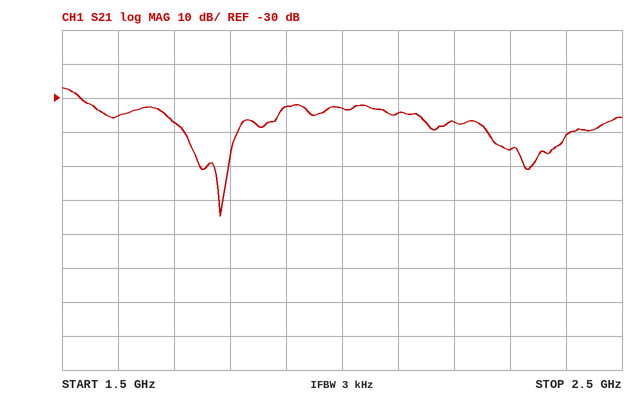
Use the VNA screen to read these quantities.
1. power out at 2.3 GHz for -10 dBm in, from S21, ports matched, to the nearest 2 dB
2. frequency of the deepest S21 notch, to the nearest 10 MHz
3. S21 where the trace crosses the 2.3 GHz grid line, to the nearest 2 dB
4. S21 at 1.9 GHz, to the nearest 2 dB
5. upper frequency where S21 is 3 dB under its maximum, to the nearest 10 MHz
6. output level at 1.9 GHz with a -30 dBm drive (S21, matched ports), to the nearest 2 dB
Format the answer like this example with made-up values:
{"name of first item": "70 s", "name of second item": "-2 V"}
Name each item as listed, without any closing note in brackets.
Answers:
{"power out at 2.3 GHz for -10 dBm in, from S21, ports matched, to the nearest 2 dB": "-56 dBm", "frequency of the deepest S21 notch, to the nearest 10 MHz": "1.78 GHz", "S21 where the trace crosses the 2.3 GHz grid line, to the nearest 2 dB": "-46 dB", "S21 at 1.9 GHz, to the nearest 2 dB": "-32 dB", "upper frequency where S21 is 3 dB under its maximum, to the nearest 10 MHz": "1.53 GHz", "output level at 1.9 GHz with a -30 dBm drive (S21, matched ports), to the nearest 2 dB": "-62 dBm"}
